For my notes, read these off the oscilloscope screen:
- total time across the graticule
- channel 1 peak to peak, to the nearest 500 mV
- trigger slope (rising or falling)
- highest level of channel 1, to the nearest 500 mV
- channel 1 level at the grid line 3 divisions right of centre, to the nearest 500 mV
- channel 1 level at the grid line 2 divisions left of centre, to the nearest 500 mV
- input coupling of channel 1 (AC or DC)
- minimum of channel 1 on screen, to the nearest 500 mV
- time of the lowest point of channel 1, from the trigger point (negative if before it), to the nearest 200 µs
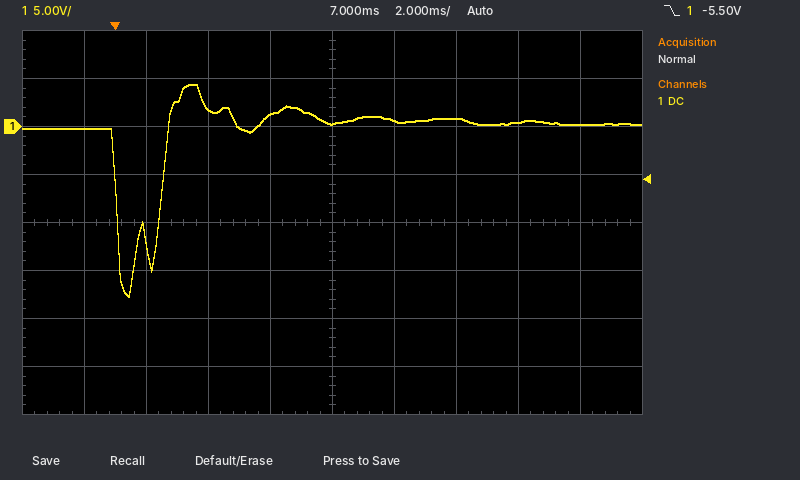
20 ms
22.0 V
falling
4.5 V
500 mV
2.0 V
DC
-17.5 V
+400 µs
